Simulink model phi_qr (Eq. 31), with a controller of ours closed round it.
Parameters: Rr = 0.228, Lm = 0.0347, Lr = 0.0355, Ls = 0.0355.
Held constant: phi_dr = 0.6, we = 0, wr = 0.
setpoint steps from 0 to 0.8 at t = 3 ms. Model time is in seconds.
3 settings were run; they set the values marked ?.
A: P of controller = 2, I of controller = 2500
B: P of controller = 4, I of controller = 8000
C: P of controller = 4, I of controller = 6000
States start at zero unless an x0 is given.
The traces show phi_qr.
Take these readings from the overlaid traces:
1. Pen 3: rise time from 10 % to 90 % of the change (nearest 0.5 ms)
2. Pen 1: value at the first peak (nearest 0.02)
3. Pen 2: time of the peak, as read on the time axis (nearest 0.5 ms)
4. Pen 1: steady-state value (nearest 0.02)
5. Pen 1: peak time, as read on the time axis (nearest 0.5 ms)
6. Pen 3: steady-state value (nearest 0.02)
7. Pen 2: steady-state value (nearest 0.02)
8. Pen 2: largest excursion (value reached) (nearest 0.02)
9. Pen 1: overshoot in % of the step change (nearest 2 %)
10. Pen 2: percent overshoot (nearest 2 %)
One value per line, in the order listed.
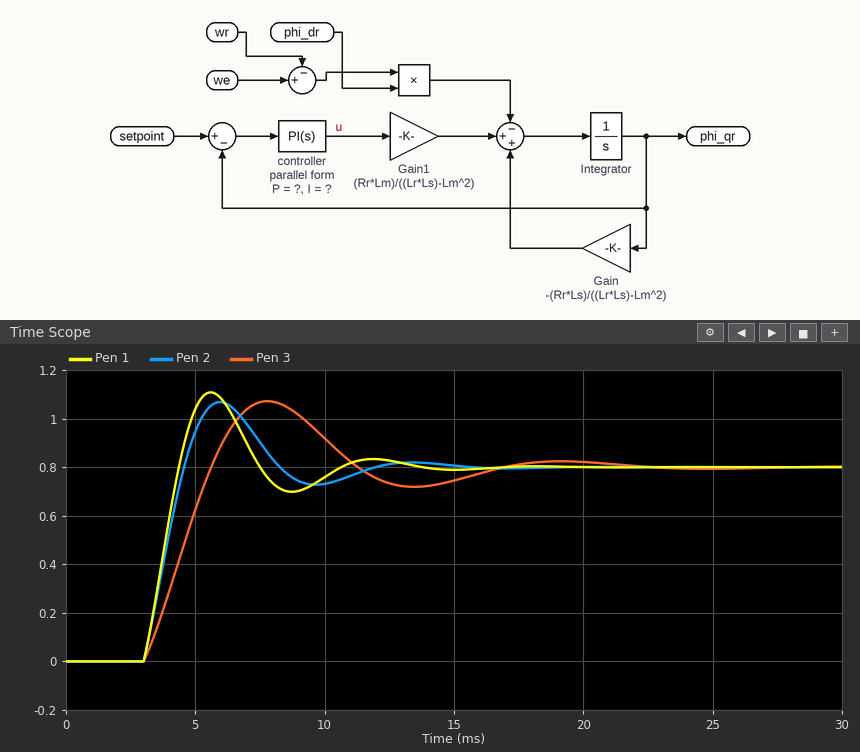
2.0 ms
1.10
6.0 ms
0.80
5.5 ms
0.80
0.80
1.06
38 %
34 %
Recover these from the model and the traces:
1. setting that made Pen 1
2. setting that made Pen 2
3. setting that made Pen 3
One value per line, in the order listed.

B
C
A
